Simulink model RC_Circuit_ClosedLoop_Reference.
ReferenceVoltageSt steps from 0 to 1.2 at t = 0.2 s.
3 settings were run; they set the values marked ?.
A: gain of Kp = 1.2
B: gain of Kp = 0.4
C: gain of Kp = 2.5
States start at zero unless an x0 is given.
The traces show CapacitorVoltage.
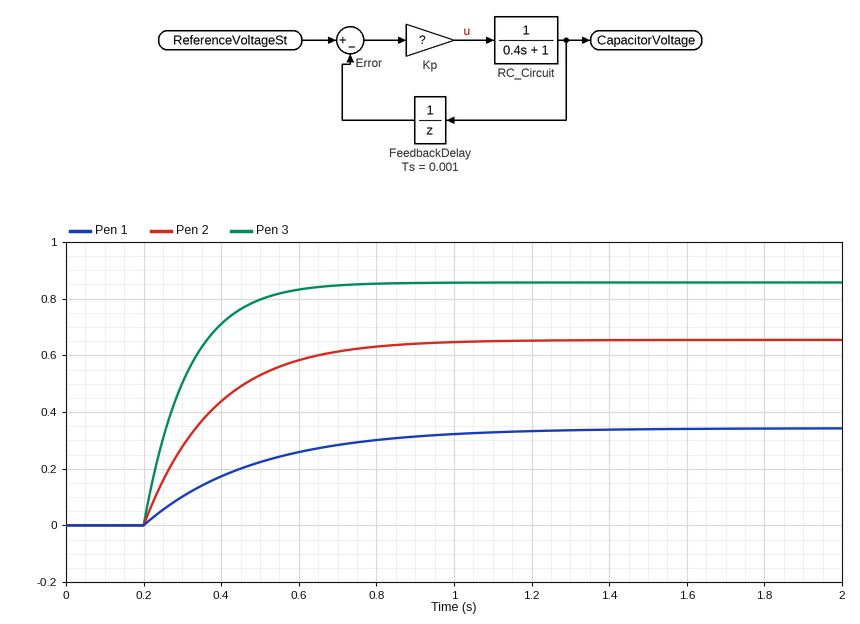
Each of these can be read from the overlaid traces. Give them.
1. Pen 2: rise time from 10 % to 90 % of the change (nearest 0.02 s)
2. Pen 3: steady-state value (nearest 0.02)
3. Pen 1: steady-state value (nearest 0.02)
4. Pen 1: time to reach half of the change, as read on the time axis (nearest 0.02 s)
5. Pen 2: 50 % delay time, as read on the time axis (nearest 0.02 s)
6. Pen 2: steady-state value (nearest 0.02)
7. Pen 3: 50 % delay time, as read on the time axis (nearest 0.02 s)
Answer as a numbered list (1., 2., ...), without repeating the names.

1. 0.40 s
2. 0.86
3. 0.34
4. 0.40 s
5. 0.32 s
6. 0.66
7. 0.28 s
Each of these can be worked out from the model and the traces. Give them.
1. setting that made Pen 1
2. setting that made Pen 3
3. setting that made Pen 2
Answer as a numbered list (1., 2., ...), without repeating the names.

1. B
2. C
3. A
